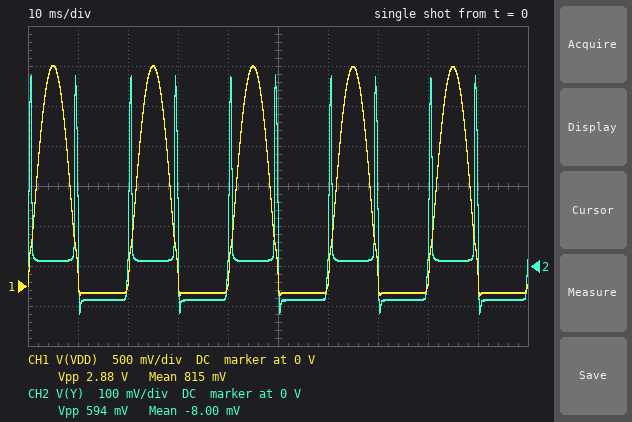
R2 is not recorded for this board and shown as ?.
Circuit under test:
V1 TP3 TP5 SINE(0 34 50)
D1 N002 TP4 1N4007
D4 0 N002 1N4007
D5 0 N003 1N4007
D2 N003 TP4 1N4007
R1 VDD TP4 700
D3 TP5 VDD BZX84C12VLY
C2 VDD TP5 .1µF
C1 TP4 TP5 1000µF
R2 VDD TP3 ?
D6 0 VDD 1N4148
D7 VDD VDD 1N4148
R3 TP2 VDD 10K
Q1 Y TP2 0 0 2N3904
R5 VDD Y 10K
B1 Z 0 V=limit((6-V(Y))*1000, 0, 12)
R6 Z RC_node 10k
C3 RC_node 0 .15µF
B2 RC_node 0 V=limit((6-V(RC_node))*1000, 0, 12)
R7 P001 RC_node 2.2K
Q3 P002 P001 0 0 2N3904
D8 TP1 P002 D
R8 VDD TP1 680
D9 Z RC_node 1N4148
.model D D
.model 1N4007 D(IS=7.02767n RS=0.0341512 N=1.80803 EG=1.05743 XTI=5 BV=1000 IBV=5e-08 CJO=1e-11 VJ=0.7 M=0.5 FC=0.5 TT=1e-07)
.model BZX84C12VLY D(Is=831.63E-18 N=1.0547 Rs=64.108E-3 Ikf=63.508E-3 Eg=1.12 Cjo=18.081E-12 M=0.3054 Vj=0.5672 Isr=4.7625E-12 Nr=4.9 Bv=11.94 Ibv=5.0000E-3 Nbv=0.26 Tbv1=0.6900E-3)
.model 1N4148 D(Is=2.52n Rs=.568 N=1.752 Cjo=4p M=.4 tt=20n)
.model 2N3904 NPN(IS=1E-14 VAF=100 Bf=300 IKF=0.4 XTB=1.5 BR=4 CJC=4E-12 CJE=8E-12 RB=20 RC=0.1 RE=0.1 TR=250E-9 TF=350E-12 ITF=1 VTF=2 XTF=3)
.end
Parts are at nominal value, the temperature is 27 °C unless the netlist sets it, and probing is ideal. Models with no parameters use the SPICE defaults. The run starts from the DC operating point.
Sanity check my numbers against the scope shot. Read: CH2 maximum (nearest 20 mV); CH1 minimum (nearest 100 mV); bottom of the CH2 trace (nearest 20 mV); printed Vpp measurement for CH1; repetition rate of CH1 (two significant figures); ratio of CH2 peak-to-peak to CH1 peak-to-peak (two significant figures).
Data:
480 mV
-100 mV
-120 mV
2.88 V
50 Hz
0.21
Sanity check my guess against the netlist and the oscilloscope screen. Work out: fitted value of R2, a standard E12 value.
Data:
3.3 kΩ
